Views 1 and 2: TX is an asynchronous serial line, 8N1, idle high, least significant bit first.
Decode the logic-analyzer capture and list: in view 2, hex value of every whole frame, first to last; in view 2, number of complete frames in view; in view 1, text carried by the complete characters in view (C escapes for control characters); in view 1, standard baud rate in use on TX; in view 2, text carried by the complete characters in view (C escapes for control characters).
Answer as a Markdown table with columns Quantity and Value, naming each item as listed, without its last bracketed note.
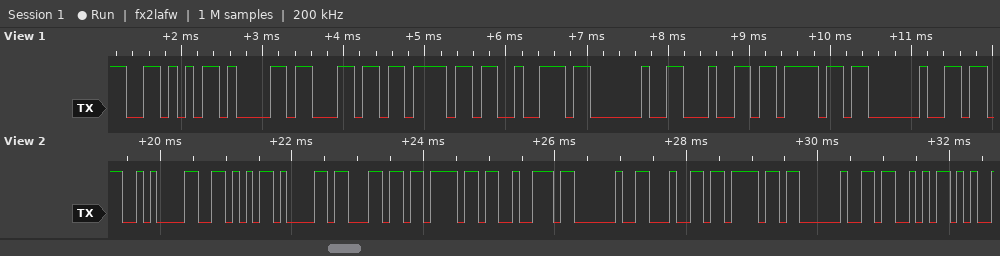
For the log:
| Quantity | Value |
|---|---|
| in view 2, hex value of every whole frame, first to last | 0A 56 61 6C 6F 72 20 64 6F 20 53 |
| in view 2, number of complete frames in view | 11 |
| in view 1, text carried by the complete characters in view | "Valor do " |
| in view 1, standard baud rate in use on TX | 9600 baud |
| in view 2, text carried by the complete characters in view | "\nValor do S" |
